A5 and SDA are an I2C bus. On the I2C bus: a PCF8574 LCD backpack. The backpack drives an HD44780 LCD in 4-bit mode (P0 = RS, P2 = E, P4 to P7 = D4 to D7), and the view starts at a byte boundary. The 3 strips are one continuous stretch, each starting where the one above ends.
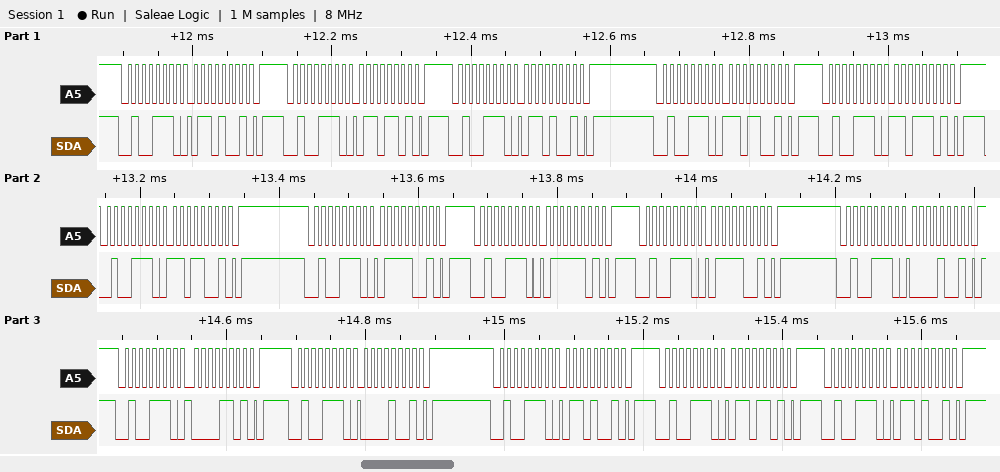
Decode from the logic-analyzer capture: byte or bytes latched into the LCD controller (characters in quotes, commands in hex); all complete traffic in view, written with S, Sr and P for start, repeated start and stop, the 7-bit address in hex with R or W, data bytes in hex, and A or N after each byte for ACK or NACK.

'm' 'p'
S 27W A 69 A P S 27W A 6D A P S 27W A 69 A P S 27W A D9 A P S 27W A DD A P S 27W A D9 A P S 27W A 79 A P S 27W A 7D A P S 27W A 79 A P S 27W A 09 A P S 27W A 0D A P S 27W A 09 A P S 27W A 69 A P S 27W A 6D A P S 27W A 69 A P
